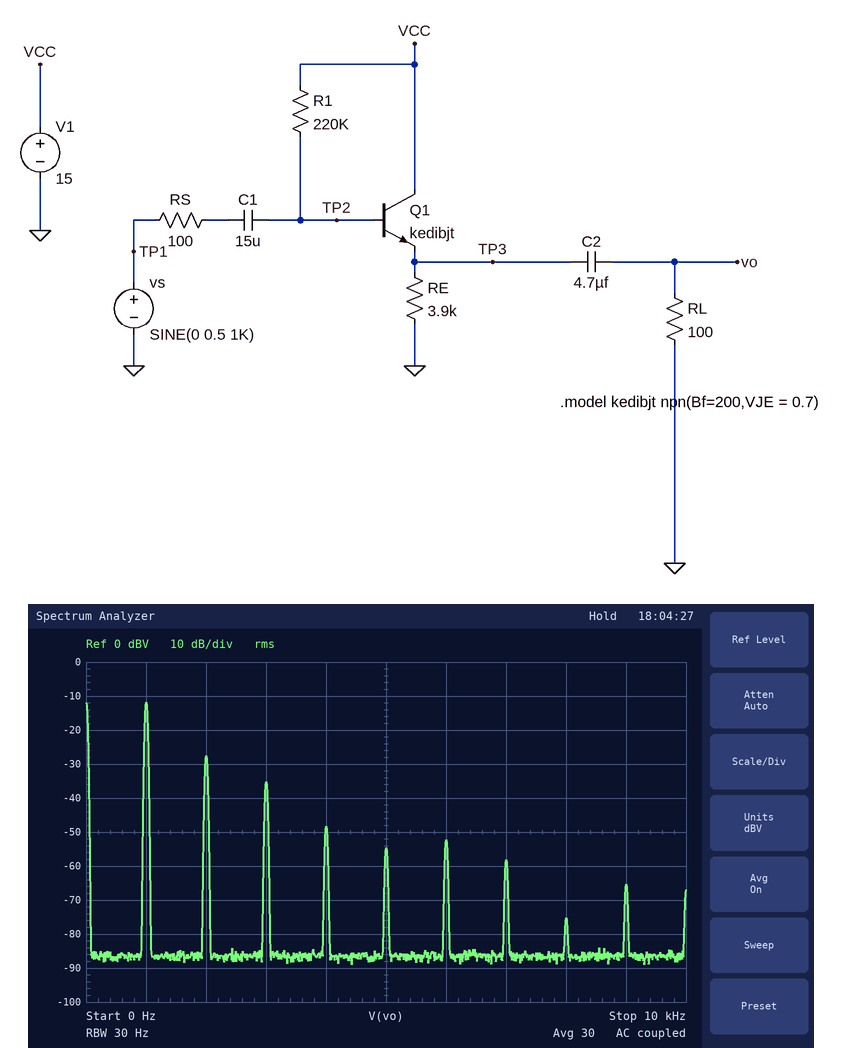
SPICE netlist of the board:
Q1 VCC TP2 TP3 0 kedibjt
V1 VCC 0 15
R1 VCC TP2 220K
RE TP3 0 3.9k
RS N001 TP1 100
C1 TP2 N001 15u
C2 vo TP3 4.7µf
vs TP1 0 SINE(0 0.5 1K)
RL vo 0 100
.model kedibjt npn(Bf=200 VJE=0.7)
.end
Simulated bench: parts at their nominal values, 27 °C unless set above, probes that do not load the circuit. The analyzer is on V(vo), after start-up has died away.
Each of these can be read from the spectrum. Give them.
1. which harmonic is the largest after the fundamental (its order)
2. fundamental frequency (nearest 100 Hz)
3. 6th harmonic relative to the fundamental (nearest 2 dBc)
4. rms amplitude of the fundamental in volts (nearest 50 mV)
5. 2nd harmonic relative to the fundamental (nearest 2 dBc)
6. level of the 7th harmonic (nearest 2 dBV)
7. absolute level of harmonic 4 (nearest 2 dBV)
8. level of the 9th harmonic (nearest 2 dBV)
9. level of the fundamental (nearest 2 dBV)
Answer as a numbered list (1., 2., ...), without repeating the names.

1. 2
2. 1.0 kHz
3. -40 dBc
4. 250 mV
5. -16 dBc
6. -58 dBV
7. -48 dBV
8. -66 dBV
9. -12 dBV
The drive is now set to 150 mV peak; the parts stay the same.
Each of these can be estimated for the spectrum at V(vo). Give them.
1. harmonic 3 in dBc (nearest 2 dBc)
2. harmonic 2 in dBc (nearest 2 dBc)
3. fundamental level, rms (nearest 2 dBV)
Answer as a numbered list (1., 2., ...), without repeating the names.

1. -56 dBc
2. -40 dBc
3. -20 dBV
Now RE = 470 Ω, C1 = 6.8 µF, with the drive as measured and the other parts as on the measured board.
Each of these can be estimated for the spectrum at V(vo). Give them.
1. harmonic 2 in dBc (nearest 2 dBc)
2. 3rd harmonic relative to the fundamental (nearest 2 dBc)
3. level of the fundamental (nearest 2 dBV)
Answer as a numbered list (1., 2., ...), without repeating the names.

1. -44 dBc
2. -58 dBc
3. -10 dBV
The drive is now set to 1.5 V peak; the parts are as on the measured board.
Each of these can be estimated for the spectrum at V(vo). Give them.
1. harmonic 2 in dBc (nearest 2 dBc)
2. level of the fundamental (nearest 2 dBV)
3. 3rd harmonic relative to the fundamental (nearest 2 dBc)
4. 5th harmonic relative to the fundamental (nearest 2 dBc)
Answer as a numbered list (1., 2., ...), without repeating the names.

1. -6 dBc
2. -10 dBV
3. -18 dBc
4. -24 dBc
